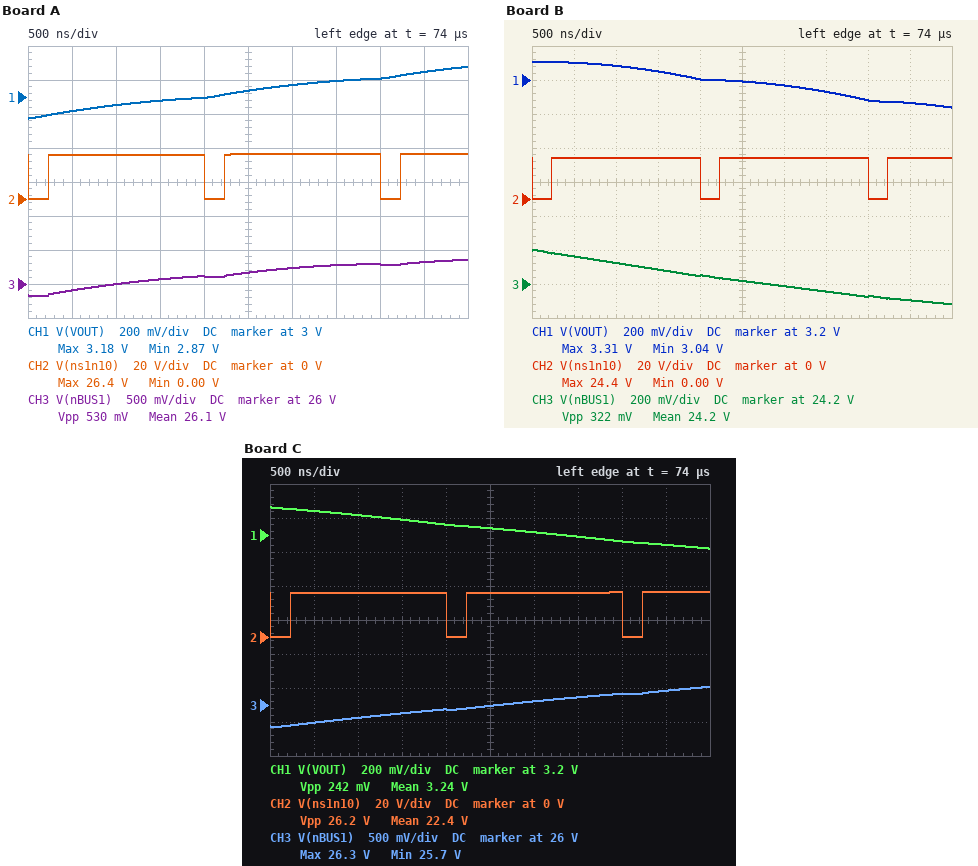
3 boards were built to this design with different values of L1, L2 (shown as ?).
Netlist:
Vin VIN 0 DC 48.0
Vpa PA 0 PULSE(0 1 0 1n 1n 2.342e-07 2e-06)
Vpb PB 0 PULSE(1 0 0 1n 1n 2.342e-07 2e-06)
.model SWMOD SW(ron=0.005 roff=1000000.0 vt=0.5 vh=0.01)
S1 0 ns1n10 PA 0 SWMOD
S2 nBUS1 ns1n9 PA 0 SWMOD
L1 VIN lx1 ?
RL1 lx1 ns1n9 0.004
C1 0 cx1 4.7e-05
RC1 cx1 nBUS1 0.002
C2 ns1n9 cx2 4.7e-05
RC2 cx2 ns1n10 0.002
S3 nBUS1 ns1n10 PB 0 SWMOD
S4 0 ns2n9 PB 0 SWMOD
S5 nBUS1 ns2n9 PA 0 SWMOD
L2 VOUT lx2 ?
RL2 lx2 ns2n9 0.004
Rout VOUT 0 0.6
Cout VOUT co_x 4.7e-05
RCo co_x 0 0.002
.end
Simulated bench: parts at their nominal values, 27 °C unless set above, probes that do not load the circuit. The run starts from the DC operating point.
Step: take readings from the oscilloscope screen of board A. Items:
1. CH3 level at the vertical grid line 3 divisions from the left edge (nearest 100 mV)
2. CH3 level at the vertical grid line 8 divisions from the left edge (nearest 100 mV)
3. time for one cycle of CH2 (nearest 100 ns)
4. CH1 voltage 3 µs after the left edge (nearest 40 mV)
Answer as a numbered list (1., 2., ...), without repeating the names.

1. 26.1 V
2. 26.3 V
3. 2.0 µs
4. 3.08 V
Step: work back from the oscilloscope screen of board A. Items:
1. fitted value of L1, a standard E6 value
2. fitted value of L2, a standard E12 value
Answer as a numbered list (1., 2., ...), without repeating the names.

1. 1 µH
2. 1.8 µH
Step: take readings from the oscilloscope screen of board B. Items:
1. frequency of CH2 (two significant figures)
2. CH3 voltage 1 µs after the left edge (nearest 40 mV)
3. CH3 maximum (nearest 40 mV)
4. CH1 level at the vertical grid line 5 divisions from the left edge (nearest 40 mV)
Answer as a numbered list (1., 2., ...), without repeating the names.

1. 500 kHz
2. 24.32 V
3. 24.40 V
4. 3.20 V
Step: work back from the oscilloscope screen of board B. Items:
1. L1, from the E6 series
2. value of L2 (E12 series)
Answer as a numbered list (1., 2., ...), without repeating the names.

1. 6.8 µH
2. 1.2 µH
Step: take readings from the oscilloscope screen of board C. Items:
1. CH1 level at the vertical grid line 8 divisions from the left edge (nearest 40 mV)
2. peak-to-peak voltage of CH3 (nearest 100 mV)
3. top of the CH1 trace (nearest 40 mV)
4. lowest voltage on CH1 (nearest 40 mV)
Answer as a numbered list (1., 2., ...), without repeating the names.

1. 3.16 V
2. 600 mV
3. 3.36 V
4. 3.12 V
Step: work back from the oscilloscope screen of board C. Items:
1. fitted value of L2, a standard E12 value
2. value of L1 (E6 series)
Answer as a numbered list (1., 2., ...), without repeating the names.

1. 5.6 µH
2. 3.3 µH
